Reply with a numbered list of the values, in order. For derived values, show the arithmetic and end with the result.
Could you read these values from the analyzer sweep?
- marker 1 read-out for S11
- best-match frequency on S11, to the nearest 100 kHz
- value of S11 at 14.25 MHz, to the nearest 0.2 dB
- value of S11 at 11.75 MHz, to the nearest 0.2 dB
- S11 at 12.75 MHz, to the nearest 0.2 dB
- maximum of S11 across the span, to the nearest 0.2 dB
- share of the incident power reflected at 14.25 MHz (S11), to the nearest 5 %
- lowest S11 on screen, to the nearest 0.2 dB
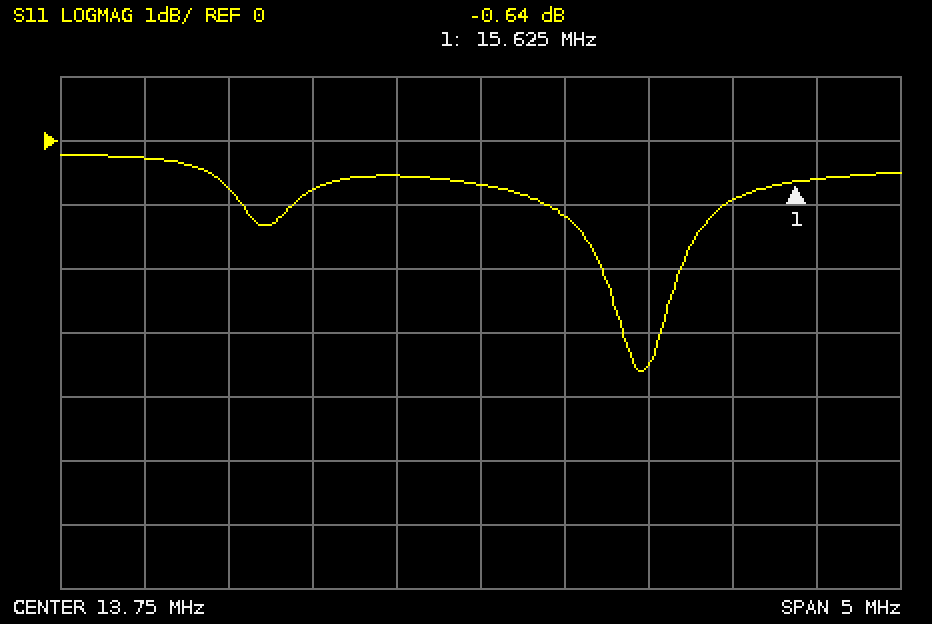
1. -0.64 dB
2. 14.7 MHz
3. -1.2 dB
4. -0.2 dB
5. -0.8 dB
6. -0.2 dB
7. 10^(-1.2/10) ≈ 75.9 %, so 75 % to the nearest 5 %
8. -3.6 dB
